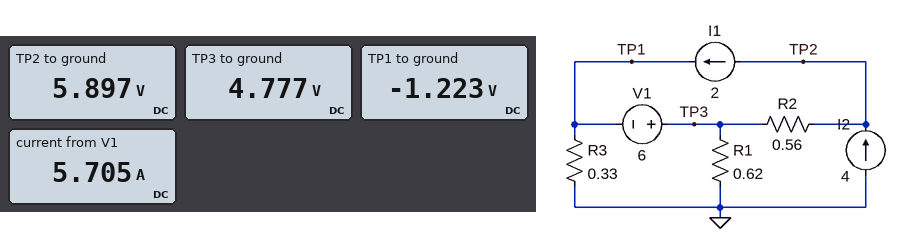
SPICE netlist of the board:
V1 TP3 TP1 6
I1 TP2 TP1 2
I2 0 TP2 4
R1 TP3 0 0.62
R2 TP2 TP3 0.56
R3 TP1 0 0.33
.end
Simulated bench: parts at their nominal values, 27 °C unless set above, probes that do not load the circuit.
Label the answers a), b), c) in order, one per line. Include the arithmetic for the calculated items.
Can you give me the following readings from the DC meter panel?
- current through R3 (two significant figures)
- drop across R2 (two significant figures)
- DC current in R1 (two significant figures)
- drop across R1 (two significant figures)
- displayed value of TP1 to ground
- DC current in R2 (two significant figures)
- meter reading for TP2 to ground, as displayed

a) (0 V - (-1.223 V)) / 330 mΩ = 3.7 A
b) 5.897 V - 4.777 V = 1.1 V
c) (4.777 V) / 620 mΩ = 7.7 A
d) 4.777 V = 4.8 V
e) -1.223 V
f) (5.897 V - 4.777 V) / 560 mΩ = 2.0 A
g) 5.897 V
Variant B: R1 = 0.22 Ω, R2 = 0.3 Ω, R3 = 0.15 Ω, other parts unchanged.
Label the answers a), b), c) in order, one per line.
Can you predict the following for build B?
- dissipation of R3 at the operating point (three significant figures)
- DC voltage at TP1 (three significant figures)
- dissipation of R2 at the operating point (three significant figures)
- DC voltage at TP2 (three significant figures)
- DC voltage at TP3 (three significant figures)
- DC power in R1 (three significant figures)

a) 28.7 W
b) -2.08 V
c) 1.20 W
d) 4.52 V
e) 3.92 V
f) 70.0 W
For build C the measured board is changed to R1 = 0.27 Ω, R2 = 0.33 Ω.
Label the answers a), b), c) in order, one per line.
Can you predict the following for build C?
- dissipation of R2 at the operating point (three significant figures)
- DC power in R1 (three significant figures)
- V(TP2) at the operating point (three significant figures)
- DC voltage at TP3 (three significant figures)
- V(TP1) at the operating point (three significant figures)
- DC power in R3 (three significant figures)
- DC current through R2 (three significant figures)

a) 1.32 W
b) 40.2 W
c) 3.95 V
d) 3.29 V
e) -2.71 V
f) 22.2 W
g) 2.00 A
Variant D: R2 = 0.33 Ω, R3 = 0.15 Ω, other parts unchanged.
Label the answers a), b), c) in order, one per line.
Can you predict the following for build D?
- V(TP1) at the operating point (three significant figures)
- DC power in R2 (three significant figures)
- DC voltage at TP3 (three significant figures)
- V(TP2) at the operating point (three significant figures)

a) -686 mV
b) 1.32 W
c) 5.31 V
d) 5.97 V
